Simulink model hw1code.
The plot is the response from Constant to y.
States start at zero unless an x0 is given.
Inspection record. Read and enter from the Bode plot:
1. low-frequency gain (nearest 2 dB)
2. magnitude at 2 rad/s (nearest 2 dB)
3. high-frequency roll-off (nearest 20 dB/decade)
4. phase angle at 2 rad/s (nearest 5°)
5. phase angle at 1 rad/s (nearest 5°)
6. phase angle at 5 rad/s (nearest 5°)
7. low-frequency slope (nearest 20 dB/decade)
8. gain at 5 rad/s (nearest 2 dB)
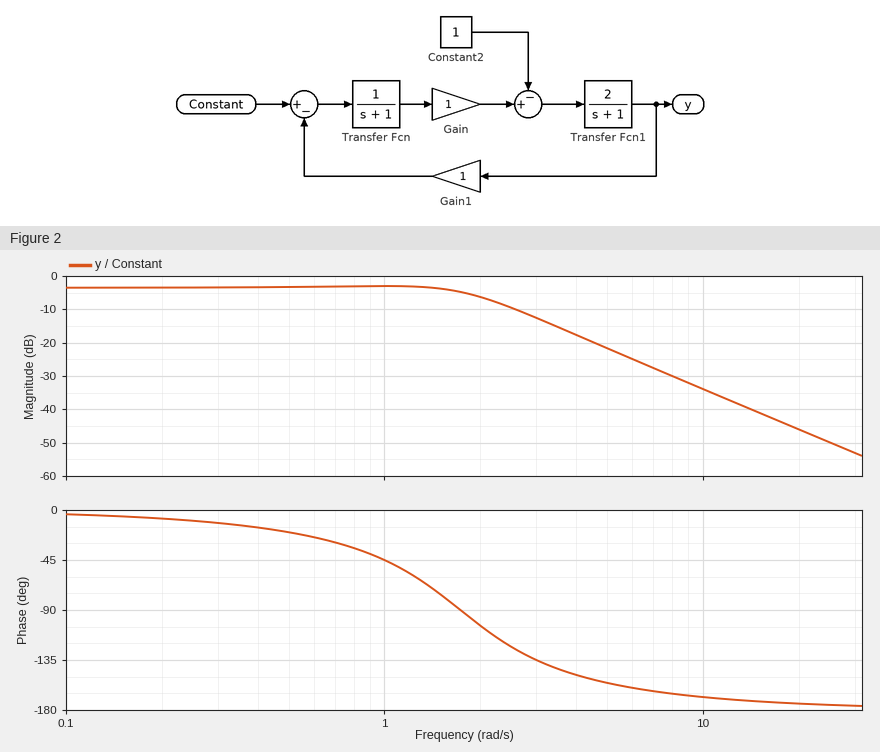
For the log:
-4 dB
-6 dB
-40 dB/decade
-105°
-45°
-155°
0 dB/decade
-22 dB
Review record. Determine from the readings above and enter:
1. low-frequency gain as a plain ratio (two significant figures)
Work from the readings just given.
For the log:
0.63
